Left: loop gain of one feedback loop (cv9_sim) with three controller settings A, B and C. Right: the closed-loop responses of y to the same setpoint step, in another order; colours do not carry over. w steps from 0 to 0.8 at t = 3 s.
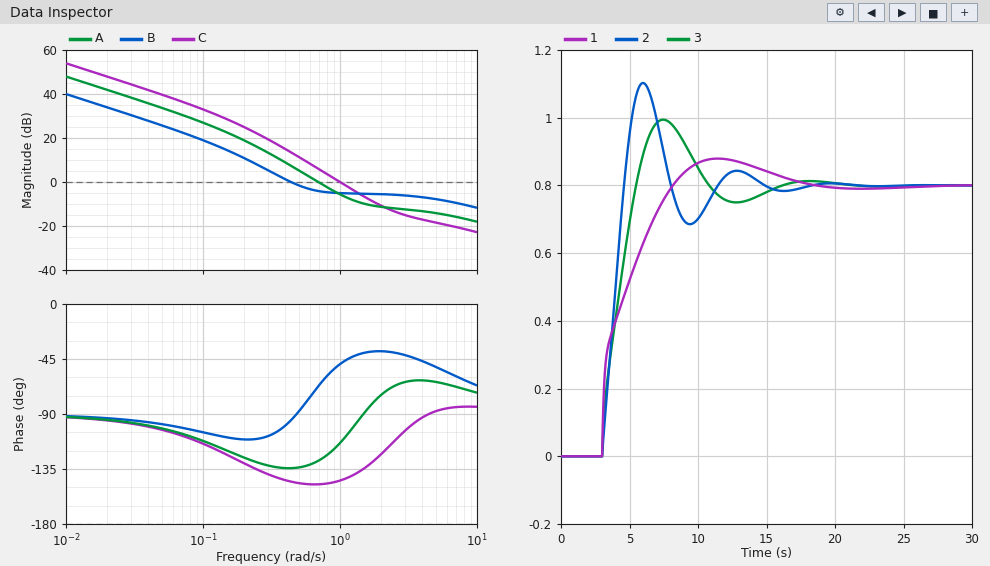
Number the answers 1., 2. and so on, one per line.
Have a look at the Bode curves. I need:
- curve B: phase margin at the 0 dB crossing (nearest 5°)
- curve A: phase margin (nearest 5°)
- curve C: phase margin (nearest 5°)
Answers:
1. 85°
2. 50°
3. 35°
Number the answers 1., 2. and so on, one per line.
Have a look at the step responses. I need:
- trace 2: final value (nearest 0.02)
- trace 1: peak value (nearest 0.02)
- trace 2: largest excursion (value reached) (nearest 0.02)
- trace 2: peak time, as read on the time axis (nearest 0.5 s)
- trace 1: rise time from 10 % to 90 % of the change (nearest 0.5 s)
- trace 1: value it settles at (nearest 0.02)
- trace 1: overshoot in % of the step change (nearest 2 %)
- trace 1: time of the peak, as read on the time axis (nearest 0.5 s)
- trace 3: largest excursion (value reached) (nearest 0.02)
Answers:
1. 0.80
2. 0.88
3. 1.10
4. 6.0 s
5. 4.0 s
6. 0.80
7. 10 %
8. 11.5 s
9. 1.00
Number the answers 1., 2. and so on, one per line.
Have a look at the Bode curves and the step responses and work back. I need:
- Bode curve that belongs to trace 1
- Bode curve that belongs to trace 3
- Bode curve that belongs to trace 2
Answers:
1. B
2. A
3. C
